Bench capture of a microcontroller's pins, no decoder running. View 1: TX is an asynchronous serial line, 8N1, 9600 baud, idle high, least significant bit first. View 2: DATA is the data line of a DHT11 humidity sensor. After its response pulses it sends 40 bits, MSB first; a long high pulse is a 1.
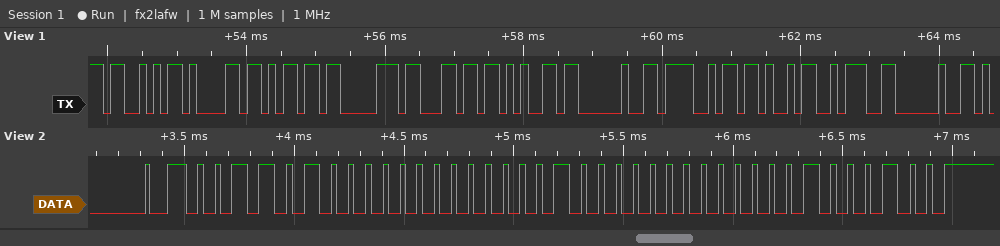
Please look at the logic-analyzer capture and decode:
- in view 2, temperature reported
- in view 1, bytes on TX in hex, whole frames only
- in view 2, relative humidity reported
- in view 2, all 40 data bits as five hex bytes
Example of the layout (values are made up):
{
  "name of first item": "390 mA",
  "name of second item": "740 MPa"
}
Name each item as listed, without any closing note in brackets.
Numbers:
{
  "in view 2, temperature reported": "16.0 °C",
  "in view 1, bytes on TX in hex, whole frames only": "0x53 0x61 0x6D 0x70 0x6C 0x65 0x20 0x4F 0x4B 0x3A 0x20",
  "in view 2, relative humidity reported": "52 %",
  "in view 2, all 40 data bits as five hex bytes": "34 00 10 00 44"
}
